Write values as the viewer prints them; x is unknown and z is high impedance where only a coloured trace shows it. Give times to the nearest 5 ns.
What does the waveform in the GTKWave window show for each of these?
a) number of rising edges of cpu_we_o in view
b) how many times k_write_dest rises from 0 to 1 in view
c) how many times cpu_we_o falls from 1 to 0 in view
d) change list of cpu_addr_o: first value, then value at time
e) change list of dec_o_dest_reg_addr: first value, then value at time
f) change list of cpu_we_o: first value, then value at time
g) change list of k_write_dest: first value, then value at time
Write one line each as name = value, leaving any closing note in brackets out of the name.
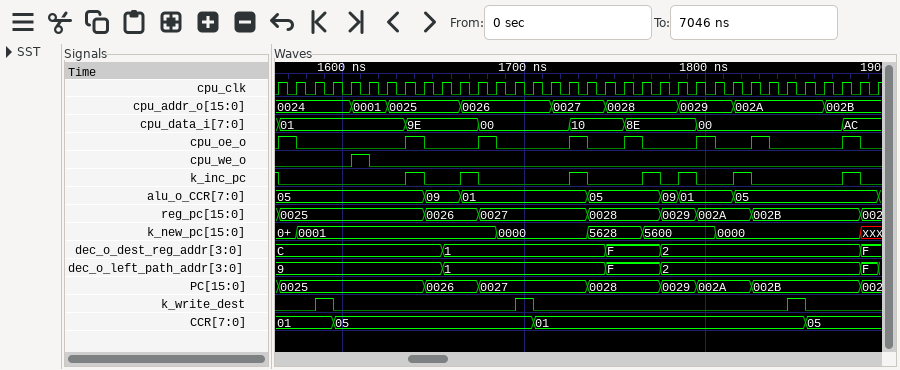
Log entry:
number of rising edges of cpu_we_o in view = 1
how many times k_write_dest rises from 0 to 1 in view = 3
how many times cpu_we_o falls from 1 to 0 in view = 1
change list of cpu_addr_o: first value, then value at time = 0024, 0001 at 1605 ns, 0025 at 1625 ns, 0026 at 1665 ns, 0027 at 1715 ns, 0028 at 1745 ns, 0029 at 1785 ns, 002A at 1815 ns, 002B at 1865 ns
change list of dec_o_dest_reg_addr: first value, then value at time = C, 1 at 1655 ns, F at 1745 ns, 2 at 1775 ns, F at 1885 ns
change list of cpu_we_o: first value, then value at time = 0, 1 at 1605 ns, 0 at 1615 ns
change list of k_write_dest: first value, then value at time = 0, 1 at 1585 ns, 0 at 1595 ns, 1 at 1695 ns, 0 at 1705 ns, 1 at 1845 ns, 0 at 1855 ns
